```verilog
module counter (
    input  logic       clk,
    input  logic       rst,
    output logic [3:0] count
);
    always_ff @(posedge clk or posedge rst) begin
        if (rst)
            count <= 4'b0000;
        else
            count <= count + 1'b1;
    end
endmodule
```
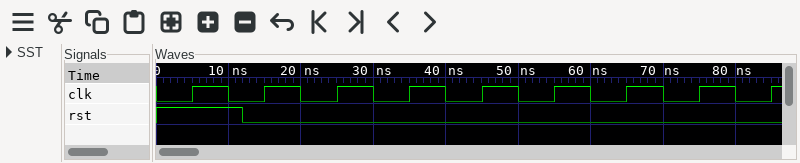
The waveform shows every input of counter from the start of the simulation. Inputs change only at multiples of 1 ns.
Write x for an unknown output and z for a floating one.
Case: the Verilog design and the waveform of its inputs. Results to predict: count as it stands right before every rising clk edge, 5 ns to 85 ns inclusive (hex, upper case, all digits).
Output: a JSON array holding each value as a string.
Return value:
["0, 0, 1, 2, 3, 4, 5, 6, 7"]
